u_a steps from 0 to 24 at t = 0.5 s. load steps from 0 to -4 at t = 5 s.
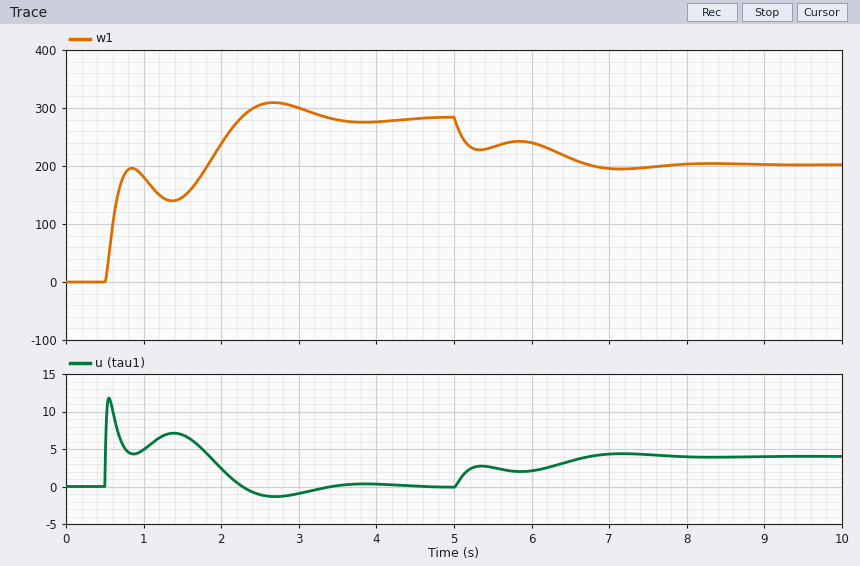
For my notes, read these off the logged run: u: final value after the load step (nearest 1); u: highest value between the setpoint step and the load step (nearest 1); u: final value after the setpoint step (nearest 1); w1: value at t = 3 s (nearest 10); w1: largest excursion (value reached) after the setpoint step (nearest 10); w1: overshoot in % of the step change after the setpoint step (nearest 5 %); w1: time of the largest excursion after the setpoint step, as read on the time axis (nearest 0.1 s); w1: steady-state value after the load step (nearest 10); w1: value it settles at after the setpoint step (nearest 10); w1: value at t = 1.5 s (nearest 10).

4
12
0
300
310
10 %
2.7 s
200
280
150
